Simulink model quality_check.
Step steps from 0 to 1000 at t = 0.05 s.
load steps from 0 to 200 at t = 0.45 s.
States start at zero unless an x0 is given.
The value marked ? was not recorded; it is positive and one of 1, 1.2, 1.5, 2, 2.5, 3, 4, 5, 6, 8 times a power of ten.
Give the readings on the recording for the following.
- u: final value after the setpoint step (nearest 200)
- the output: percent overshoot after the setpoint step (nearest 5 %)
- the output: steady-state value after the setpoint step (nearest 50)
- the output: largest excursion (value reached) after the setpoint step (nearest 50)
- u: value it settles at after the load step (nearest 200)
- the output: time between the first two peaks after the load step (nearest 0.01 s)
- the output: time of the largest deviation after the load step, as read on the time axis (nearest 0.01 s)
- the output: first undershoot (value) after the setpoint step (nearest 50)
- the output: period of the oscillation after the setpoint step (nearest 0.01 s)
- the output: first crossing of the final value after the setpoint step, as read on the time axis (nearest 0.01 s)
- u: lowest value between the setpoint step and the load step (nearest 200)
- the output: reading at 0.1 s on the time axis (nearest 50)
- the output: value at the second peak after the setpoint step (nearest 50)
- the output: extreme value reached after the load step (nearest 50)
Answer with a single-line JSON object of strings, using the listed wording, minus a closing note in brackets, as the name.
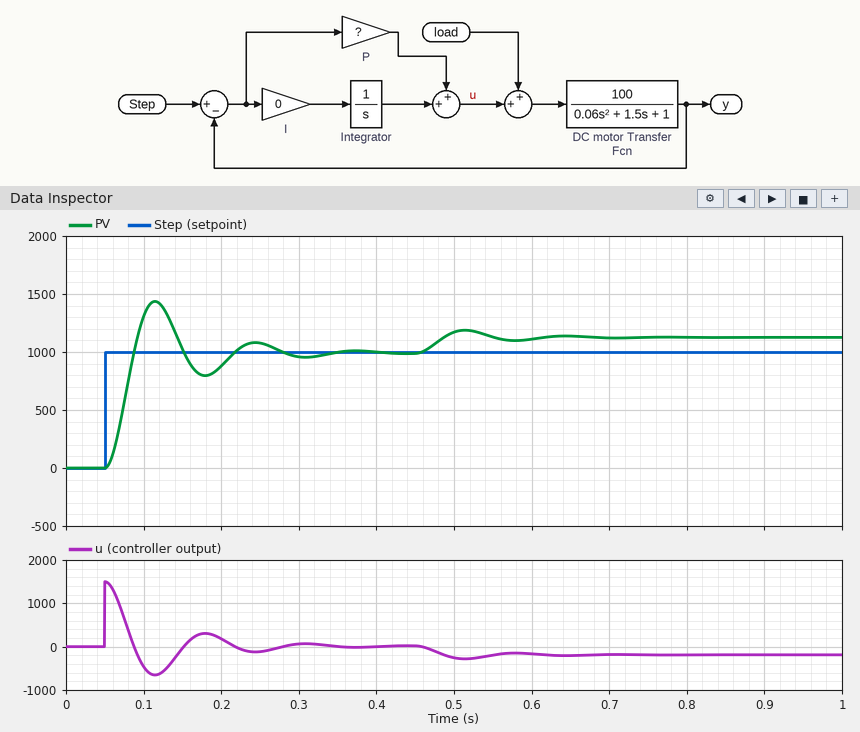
{"u: final value after the setpoint step": "0", "the output: percent overshoot after the setpoint step": "45 %", "the output: steady-state value after the setpoint step": "1000", "the output: largest excursion (value reached) after the setpoint step": "1450", "u: value it settles at after the load step": "-200", "the output: time between the first two peaks after the load step": "0.13 s", "the output: time of the largest deviation after the load step, as read on the time axis": "0.51 s", "the output: first undershoot (value) after the setpoint step": "800", "the output: period of the oscillation after the setpoint step": "0.13 s", "the output: first crossing of the final value after the setpoint step, as read on the time axis": "0.09 s", "u: lowest value between the setpoint step and the load step": "-600", "the output: reading at 0.1 s on the time axis": "1300", "the output: value at the second peak after the setpoint step": "1100", "the output: extreme value reached after the load step": "1200"}
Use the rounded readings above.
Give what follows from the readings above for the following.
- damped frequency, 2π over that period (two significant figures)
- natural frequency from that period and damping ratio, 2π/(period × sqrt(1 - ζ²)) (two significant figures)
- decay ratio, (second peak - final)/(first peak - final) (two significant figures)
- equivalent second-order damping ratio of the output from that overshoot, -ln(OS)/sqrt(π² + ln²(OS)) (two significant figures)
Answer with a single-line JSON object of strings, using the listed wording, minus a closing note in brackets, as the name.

{"damped frequency, 2π over that period": "48 rad/s", "natural frequency from that period and damping ratio, 2π/(period × sqrt(1 - ζ²))": "50 rad/s", "decay ratio, (second peak - final)/(first peak - final)": "0.22", "equivalent second-order damping ratio of the output from that overshoot, -ln(OS)/sqrt(π² + ln²(OS))": "0.25"}
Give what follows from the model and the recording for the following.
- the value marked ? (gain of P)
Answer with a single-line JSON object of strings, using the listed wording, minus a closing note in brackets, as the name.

{"the value marked ?": "1.5"}
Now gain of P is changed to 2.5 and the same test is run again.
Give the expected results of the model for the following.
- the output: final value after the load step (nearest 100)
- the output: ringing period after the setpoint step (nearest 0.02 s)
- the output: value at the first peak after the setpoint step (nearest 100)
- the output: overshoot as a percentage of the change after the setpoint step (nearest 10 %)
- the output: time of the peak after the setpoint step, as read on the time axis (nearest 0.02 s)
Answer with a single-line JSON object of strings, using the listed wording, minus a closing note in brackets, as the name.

{"the output: final value after the load step": "1100", "the output: ringing period after the setpoint step": "0.10 s", "the output: value at the first peak after the setpoint step": "1500", "the output: overshoot as a percentage of the change after the setpoint step": "50 %", "the output: time of the peak after the setpoint step, as read on the time axis": "0.10 s"}
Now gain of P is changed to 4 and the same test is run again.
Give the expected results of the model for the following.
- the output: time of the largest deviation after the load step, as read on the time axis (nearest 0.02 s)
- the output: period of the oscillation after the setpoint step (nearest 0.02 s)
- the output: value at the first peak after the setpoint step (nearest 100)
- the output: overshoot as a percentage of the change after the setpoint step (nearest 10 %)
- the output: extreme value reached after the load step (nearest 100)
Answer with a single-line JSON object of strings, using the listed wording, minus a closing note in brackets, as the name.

{"the output: time of the largest deviation after the load step, as read on the time axis": "0.48 s", "the output: period of the oscillation after the setpoint step": "0.08 s", "the output: value at the first peak after the setpoint step": "1600", "the output: overshoot as a percentage of the change after the setpoint step": "60 %", "the output: extreme value reached after the load step": "1100"}
